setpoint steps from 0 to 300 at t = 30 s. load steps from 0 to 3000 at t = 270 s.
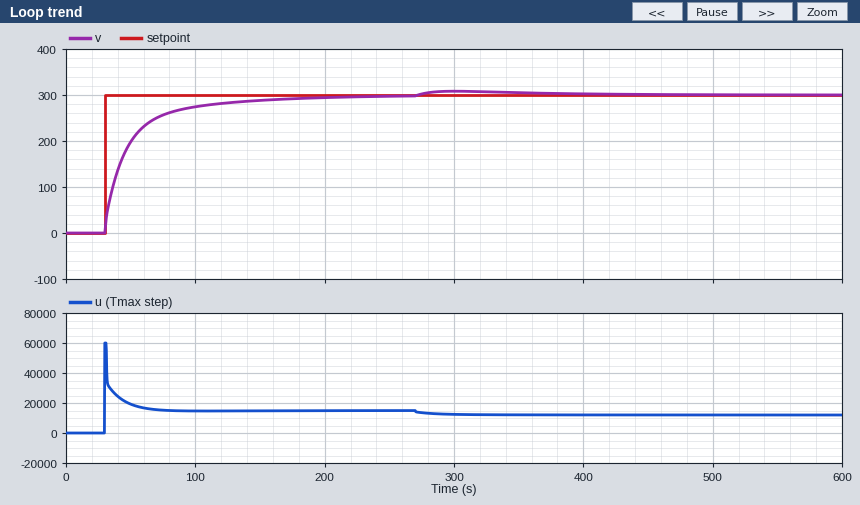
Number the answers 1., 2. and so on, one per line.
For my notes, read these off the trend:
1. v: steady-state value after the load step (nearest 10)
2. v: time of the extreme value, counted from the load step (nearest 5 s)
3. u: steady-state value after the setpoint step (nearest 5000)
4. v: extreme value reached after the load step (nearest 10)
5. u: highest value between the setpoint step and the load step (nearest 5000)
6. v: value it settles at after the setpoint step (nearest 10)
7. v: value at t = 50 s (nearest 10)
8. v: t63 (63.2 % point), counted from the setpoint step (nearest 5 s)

1. 300
2. 30 s
3. 15000
4. 310
5. 60000
6. 300
7. 200
8. 20 s
